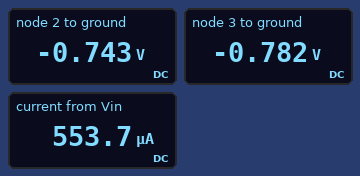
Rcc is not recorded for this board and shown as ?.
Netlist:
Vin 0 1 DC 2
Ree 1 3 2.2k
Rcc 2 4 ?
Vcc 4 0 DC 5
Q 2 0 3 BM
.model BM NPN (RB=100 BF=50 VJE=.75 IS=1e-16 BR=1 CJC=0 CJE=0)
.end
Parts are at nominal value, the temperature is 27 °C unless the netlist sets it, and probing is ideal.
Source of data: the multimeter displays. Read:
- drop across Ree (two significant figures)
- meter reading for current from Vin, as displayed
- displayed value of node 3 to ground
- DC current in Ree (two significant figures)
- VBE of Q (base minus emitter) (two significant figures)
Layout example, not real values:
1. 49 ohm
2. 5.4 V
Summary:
1. 1.2 V
2. 553.7 µA
3. -0.782 V
4. 550 µA
5. 780 mV
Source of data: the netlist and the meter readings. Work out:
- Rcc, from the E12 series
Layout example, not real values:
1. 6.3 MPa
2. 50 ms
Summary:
1. 15 kΩ
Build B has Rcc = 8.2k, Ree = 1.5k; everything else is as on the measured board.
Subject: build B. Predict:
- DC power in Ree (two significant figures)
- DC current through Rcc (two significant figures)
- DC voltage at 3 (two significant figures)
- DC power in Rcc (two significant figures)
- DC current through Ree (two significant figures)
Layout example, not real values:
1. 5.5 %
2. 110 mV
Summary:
1. 990 µW
2. 700 µA
3. -780 mV
4. 4.0 mW
5. 810 µA
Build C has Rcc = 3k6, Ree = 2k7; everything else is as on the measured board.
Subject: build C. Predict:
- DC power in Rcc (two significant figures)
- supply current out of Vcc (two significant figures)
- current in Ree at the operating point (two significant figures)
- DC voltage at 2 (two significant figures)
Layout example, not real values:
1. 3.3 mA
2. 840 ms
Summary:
1. 740 µW
2. 450 µA
3. 460 µA
4. 3.4 V
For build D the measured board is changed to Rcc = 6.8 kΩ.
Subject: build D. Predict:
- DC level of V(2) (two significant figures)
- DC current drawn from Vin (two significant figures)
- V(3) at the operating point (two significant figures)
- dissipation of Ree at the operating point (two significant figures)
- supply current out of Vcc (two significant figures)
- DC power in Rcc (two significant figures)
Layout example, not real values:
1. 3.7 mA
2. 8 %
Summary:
1. 1.2 V
2. 560 µA
3. -760 mV
4. 700 µW
5. 550 µA
6. 2.1 mW
